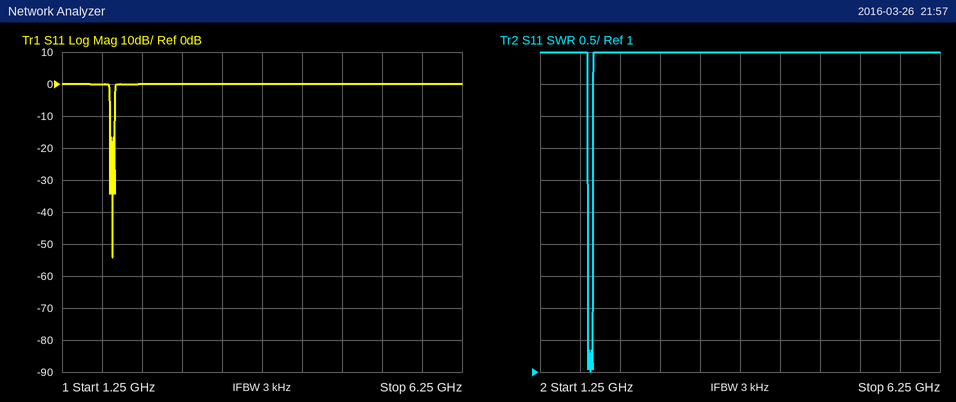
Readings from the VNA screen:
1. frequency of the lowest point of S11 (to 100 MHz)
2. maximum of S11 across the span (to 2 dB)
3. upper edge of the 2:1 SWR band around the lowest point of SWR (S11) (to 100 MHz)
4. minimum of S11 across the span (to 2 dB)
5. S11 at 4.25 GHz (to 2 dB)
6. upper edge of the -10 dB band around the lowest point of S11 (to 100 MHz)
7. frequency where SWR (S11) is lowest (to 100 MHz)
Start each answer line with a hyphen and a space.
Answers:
- 1.9 GHz
- 0 dB
- 1.9 GHz
- -54 dB
- 0 dB
- 1.9 GHz
- 1.9 GHz
